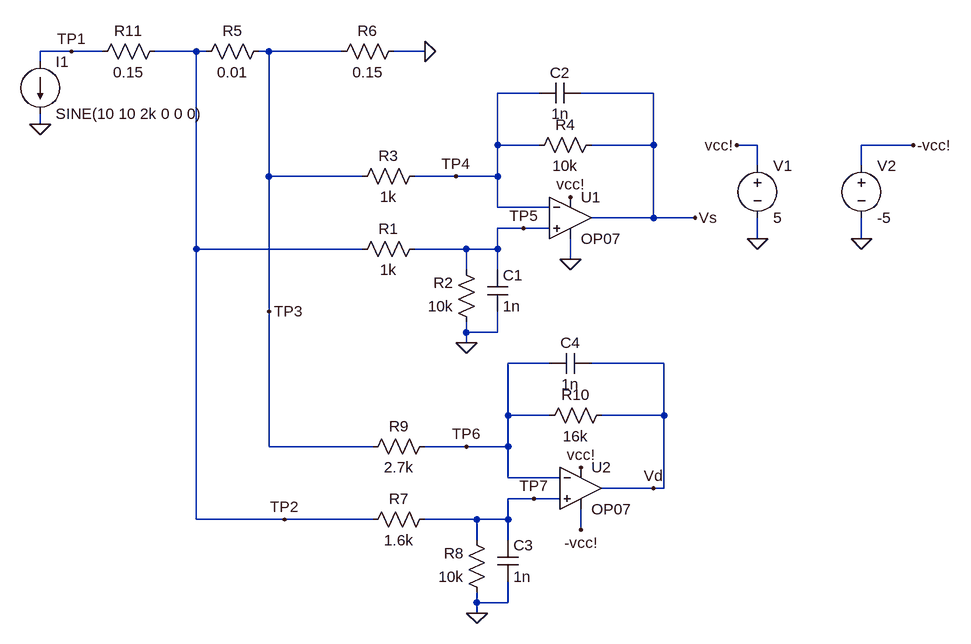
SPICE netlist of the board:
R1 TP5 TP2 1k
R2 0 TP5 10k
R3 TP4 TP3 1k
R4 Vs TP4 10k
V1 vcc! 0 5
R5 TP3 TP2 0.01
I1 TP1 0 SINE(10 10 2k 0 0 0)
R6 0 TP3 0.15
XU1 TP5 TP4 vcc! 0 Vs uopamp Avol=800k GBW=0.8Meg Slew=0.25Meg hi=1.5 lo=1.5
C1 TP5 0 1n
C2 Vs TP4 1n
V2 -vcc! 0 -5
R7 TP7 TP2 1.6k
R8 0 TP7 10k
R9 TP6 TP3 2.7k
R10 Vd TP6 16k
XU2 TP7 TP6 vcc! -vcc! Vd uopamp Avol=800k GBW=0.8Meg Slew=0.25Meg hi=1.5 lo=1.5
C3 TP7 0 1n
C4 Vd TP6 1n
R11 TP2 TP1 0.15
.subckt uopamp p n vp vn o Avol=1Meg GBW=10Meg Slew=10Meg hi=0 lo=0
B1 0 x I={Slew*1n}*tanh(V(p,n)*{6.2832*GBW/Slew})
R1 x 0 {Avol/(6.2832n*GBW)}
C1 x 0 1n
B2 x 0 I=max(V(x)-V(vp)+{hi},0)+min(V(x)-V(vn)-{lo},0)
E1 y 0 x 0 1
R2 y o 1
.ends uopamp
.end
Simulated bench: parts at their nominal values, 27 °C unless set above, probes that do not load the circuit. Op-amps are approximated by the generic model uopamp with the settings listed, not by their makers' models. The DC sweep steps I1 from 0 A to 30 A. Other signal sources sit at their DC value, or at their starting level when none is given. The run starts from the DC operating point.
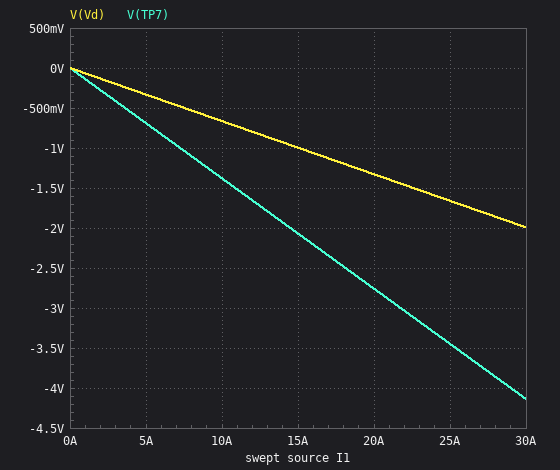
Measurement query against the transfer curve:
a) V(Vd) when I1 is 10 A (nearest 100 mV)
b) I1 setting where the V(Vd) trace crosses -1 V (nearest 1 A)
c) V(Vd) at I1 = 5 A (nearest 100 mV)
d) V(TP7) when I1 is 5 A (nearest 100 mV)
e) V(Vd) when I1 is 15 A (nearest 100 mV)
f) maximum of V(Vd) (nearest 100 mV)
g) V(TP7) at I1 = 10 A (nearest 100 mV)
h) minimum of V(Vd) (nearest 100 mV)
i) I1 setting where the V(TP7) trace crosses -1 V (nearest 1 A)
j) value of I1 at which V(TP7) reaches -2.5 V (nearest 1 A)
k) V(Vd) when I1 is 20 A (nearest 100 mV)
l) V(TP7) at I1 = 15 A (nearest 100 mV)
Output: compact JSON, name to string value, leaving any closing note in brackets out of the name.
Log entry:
{"V(Vd) when I1 is 10 A": "-700 mV", "I1 setting where the V(Vd) trace crosses -1 V": "15 A", "V(Vd) at I1 = 5 A": "-300 mV", "V(TP7) when I1 is 5 A": "-700 mV", "V(Vd) when I1 is 15 A": "-1.0 V", "maximum of V(Vd)": "0 V", "V(TP7) at I1 = 10 A": "-1.4 V", "minimum of V(Vd)": "-2.0 V", "I1 setting where the V(TP7) trace crosses -1 V": "7 A", "value of I1 at which V(TP7) reaches -2.5 V": "18 A", "V(Vd) when I1 is 20 A": "-1.3 V", "V(TP7) at I1 = 15 A": "-2.1 V"}
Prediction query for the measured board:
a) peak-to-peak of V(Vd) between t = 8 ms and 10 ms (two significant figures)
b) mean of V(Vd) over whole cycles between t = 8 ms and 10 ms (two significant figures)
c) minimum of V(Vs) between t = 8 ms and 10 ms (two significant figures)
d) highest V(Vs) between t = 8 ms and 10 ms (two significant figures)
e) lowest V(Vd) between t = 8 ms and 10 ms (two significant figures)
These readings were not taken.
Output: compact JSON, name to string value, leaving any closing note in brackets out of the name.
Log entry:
{"peak-to-peak of V(Vd) between t = 8 ms and 10 ms": "1.3 V", "mean of V(Vd) over whole cycles between t = 8 ms and 10 ms": "-660 mV", "minimum of V(Vs) between t = 8 ms and 10 ms": "1.5 V", "highest V(Vs) between t = 8 ms and 10 ms": "1.5 V", "lowest V(Vd) between t = 8 ms and 10 ms": "-1.3 V"}
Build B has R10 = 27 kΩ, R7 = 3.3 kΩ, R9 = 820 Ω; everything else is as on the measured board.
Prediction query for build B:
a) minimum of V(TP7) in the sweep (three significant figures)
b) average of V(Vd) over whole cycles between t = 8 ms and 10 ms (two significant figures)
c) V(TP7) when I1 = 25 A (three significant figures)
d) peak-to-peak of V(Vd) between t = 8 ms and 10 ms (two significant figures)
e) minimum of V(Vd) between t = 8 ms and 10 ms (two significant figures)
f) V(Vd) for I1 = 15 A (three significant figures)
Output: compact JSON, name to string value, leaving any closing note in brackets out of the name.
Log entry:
{"minimum of V(TP7) in the sweep": "-3.61 V", "average of V(Vd) over whole cycles between t = 8 ms and 10 ms": "2.9 V", "V(TP7) when I1 = 25 A": "-3.01 V", "peak-to-peak of V(Vd) between t = 8 ms and 10 ms": "3.0 V", "minimum of V(Vd) between t = 8 ms and 10 ms": "470 mV", "V(Vd) for I1 = 15 A": "3.50 V"}
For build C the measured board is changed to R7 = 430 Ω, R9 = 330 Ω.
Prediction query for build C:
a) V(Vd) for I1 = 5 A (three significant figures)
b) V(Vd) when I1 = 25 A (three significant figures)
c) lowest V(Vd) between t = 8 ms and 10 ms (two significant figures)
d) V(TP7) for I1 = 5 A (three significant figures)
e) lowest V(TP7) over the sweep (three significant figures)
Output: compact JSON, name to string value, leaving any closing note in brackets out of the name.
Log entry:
{"V(Vd) for I1 = 5 A": "-1.59 V", "V(Vd) when I1 = 25 A": "-3.50 V", "lowest V(Vd) between t = 8 ms and 10 ms": "-3.5 V", "V(TP7) for I1 = 5 A": "-767 mV", "lowest V(TP7) over the sweep": "-4.60 V"}
